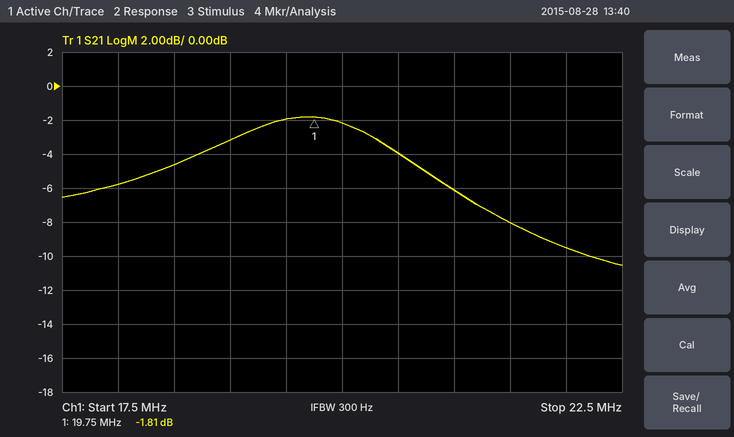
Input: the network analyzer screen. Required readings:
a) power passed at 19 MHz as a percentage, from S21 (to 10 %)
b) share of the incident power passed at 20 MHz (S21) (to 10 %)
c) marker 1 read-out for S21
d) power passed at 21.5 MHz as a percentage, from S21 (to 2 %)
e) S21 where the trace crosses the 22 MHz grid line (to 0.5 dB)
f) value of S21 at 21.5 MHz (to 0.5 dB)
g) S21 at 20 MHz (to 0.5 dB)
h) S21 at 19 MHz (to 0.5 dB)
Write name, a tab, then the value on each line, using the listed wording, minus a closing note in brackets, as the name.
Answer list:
power passed at 19 MHz as a percentage, from S21	50 %
share of the incident power passed at 20 MHz (S21)	60 %
marker 1 read-out for S21	-1.81 dB
power passed at 21.5 MHz as a percentage, from S21	16 %
S21 where the trace crosses the 22 MHz grid line	-9.5 dB
value of S21 at 21.5 MHz	-8.0 dB
S21 at 20 MHz	-2.0 dB
S21 at 19 MHz	-3.0 dB
